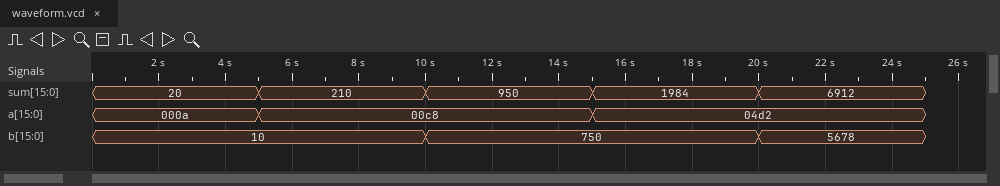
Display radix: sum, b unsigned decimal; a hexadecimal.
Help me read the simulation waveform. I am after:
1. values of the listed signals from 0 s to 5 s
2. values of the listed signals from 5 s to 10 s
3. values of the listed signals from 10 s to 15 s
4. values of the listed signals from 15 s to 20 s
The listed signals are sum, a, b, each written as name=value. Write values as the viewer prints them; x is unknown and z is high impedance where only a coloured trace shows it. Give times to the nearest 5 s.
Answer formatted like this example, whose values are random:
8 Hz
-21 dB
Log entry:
sum=20, a=000a, b=10
sum=210, a=00c8, b=10
sum=950, a=00c8, b=750
sum=1984, a=04d2, b=750
